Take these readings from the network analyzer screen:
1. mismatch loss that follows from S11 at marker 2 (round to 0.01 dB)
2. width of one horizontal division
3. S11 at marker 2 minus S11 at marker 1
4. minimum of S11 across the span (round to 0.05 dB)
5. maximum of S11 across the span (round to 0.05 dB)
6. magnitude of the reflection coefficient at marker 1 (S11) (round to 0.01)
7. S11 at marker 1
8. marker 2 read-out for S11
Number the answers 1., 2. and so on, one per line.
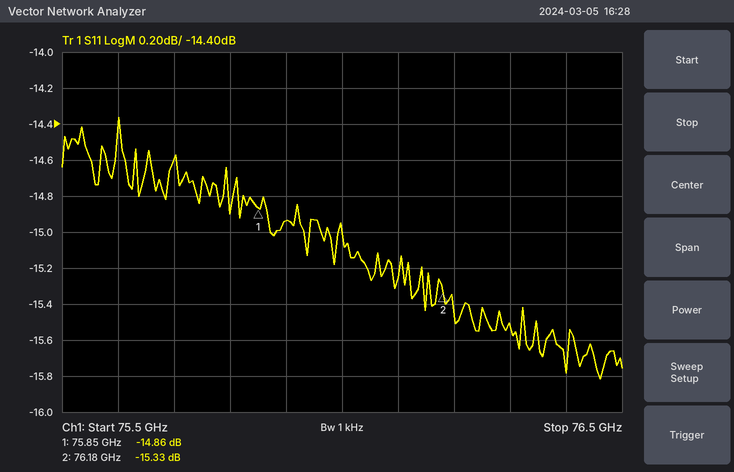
1. 0.13 dB
2. 100 MHz
3. -0.47 dB
4. -15.80 dB
5. -14.35 dB
6. 0.18
7. -14.86 dB
8. -15.33 dB
